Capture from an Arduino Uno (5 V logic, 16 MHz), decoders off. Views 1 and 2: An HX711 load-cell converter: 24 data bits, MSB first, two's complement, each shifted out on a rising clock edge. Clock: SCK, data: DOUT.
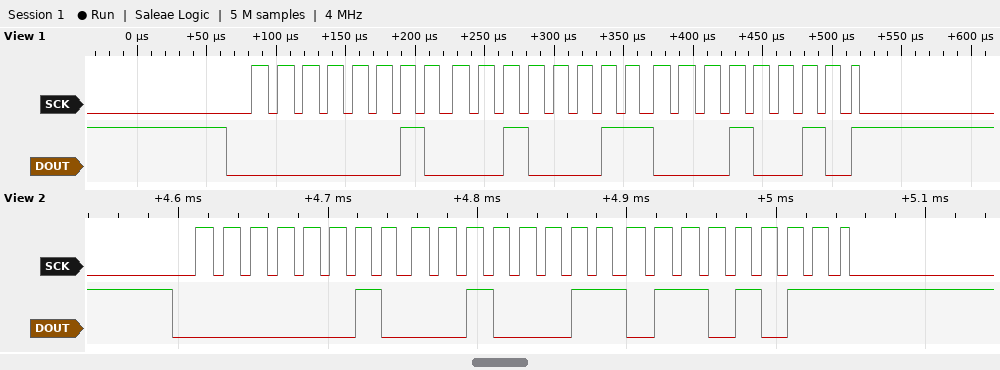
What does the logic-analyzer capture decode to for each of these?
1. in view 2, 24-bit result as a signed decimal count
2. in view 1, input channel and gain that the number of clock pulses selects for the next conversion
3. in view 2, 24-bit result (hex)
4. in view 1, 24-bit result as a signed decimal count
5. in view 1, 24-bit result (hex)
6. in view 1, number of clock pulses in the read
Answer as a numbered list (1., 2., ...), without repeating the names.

1. 140139
2. channel A, gain 128
3. 0x02236B
4. 140050
5. 0x022312
6. 25
